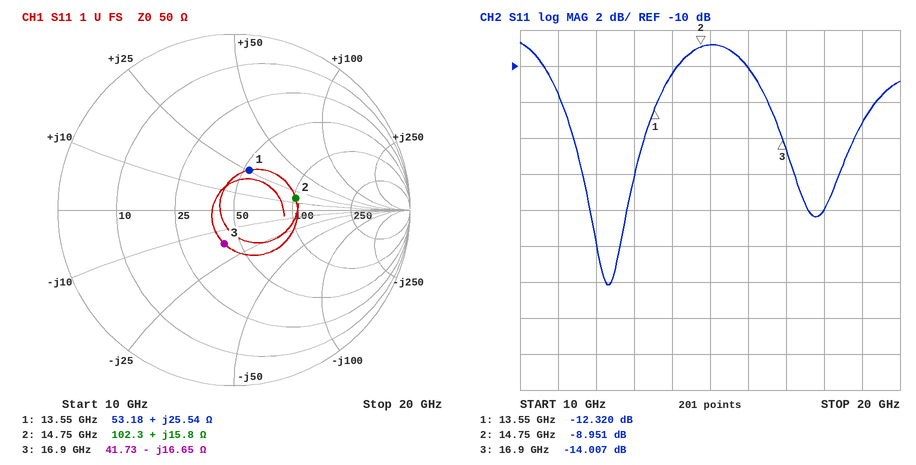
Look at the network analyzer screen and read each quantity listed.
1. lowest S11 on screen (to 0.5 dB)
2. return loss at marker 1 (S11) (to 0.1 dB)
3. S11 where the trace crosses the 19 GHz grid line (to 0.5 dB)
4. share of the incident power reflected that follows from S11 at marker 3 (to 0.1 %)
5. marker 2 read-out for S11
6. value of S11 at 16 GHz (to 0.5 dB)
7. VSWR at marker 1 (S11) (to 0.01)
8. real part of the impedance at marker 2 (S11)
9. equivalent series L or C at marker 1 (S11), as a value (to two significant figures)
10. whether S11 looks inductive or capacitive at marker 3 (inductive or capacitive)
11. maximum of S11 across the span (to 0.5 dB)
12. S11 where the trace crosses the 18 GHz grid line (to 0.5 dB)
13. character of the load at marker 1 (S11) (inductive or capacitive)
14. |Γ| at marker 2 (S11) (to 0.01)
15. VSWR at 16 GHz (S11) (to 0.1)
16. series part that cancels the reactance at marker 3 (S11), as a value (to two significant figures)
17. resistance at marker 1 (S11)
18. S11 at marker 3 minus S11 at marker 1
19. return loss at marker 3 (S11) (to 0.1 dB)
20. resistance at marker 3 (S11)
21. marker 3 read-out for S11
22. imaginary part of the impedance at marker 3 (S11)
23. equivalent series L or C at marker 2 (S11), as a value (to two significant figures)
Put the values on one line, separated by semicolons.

-22.0 dB; 12.3 dB; -13.0 dB; 4.0 %; -8.951 dB; -10.0 dB; 1.64; 102.3 Ω; 300 pH; capacitive; -8.5 dB; -18.0 dB; inductive; 0.36; 1.9; 160 pH; 53.18 Ω; -1.687 dB; 14.0 dB; 41.73 Ω; -14.007 dB; -16.65 Ω; 170 pH
